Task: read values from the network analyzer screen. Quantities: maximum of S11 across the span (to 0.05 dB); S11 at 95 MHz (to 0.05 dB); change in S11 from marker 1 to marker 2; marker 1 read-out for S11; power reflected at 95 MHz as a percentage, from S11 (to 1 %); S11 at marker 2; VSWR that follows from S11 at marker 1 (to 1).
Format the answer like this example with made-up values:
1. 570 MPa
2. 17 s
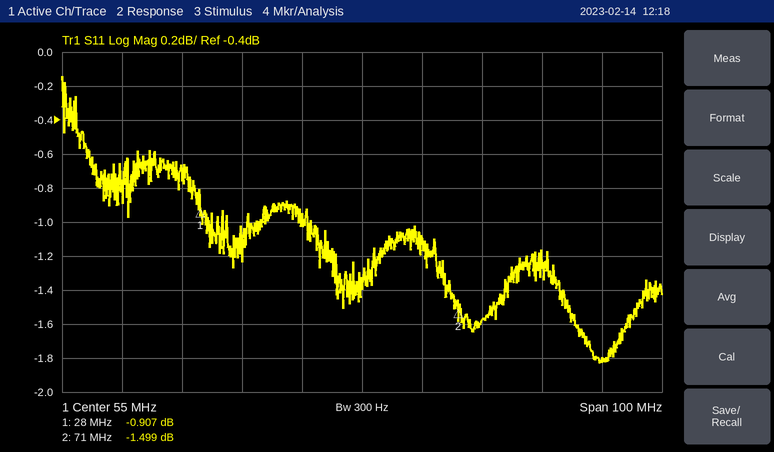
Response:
1. -0.15 dB
2. -1.80 dB
3. -0.592 dB
4. -0.907 dB
5. 66 %
6. -1.499 dB
7. 19
